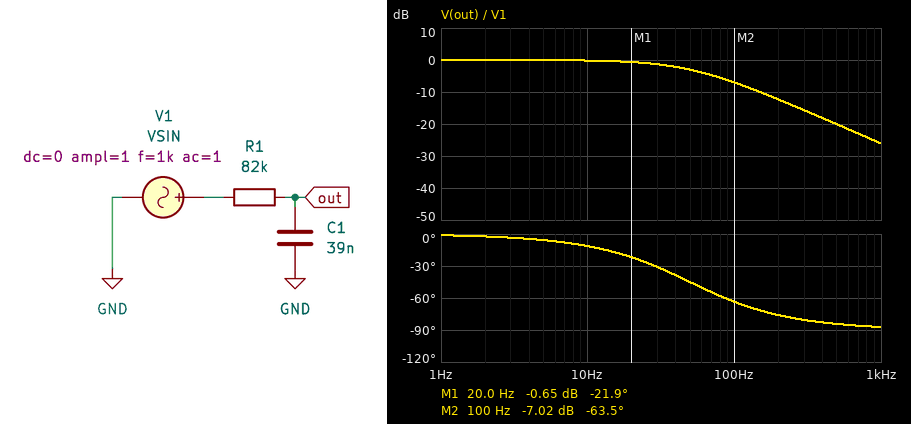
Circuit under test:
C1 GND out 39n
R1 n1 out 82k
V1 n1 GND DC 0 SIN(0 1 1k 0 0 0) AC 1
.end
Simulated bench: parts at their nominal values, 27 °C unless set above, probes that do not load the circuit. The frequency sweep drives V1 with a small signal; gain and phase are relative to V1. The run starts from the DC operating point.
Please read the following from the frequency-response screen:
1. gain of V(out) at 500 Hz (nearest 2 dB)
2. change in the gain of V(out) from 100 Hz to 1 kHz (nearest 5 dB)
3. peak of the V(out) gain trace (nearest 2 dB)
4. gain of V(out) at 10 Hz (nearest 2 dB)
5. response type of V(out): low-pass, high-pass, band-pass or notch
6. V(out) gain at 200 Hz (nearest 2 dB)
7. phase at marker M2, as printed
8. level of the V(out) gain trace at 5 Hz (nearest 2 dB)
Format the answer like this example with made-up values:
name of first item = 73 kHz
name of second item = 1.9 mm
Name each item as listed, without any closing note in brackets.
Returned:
gain of V(out) at 500 Hz = -20 dB
change in the gain of V(out) from 100 Hz to 1 kHz = -20 dB
peak of the V(out) gain trace = 0 dB
gain of V(out) at 10 Hz = 0 dB
response type of V(out): low-pass, high-pass, band-pass or notch = low-pass
V(out) gain at 200 Hz = -12 dB
phase at marker M2, as printed = -63.5 deg
level of the V(out) gain trace at 5 Hz = 0 dB
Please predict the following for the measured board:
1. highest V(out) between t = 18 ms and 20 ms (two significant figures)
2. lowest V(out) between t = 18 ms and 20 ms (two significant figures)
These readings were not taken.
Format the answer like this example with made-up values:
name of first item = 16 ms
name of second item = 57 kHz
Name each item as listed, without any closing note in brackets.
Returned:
highest V(out) between t = 18 ms and 20 ms = 50 mV
lowest V(out) between t = 18 ms and 20 ms = -50 mV
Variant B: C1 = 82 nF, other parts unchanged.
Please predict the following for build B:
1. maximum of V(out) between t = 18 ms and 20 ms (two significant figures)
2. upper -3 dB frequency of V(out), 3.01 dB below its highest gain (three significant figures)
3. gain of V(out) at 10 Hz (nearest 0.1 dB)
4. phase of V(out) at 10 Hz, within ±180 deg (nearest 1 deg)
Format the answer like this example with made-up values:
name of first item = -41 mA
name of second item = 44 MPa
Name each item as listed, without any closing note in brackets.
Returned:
maximum of V(out) between t = 18 ms and 20 ms = 25 mV
upper -3 dB frequency of V(out), 3.01 dB below its highest gain = 23.7 Hz
gain of V(out) at 10 Hz = -0.7 dB
phase of V(out) at 10 Hz, within ±180 deg = -23 deg
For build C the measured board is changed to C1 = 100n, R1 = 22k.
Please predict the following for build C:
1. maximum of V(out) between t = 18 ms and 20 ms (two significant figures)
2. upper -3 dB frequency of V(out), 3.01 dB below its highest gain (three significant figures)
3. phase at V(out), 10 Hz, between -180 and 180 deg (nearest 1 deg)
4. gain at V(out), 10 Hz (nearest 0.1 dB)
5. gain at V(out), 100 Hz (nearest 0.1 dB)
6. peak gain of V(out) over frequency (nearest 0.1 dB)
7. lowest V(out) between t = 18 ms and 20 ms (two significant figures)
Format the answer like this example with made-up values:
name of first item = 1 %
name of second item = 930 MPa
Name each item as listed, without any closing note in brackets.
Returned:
maximum of V(out) between t = 18 ms and 20 ms = 72 mV
upper -3 dB frequency of V(out), 3.01 dB below its highest gain = 72.3 Hz
phase at V(out), 10 Hz, between -180 and 180 deg = -8 deg
gain at V(out), 10 Hz = -0.1 dB
gain at V(out), 100 Hz = -4.6 dB
peak gain of V(out) over frequency = 0 dB
lowest V(out) between t = 18 ms and 20 ms = -72 mV
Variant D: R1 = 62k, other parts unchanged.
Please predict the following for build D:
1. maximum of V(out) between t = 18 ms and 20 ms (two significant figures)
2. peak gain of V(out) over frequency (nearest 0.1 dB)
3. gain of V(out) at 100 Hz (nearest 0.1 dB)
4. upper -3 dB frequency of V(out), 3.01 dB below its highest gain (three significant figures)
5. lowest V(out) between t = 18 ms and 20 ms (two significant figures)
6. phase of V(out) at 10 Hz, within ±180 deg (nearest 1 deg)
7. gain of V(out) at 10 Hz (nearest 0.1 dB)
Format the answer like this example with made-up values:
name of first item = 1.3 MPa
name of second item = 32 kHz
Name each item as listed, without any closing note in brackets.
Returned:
maximum of V(out) between t = 18 ms and 20 ms = 66 mV
peak gain of V(out) over frequency = 0 dB
gain of V(out) at 100 Hz = -5.2 dB
upper -3 dB frequency of V(out), 3.01 dB below its highest gain = 65.8 Hz
lowest V(out) between t = 18 ms and 20 ms = -66 mV
phase of V(out) at 10 Hz, within ±180 deg = -9 deg
gain of V(out) at 10 Hz = -0.1 dB
